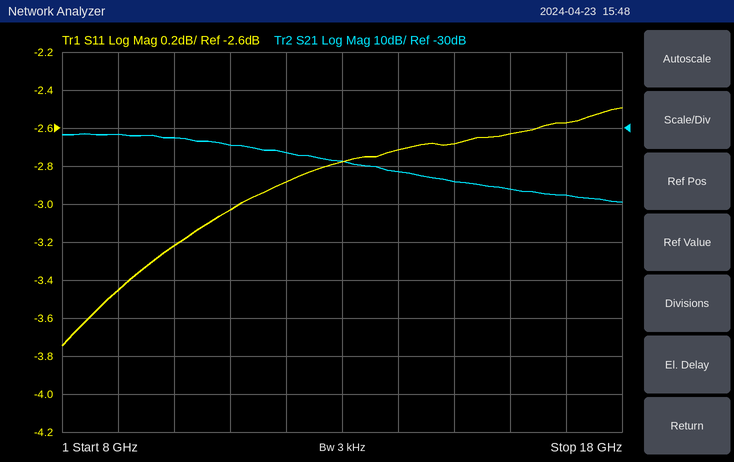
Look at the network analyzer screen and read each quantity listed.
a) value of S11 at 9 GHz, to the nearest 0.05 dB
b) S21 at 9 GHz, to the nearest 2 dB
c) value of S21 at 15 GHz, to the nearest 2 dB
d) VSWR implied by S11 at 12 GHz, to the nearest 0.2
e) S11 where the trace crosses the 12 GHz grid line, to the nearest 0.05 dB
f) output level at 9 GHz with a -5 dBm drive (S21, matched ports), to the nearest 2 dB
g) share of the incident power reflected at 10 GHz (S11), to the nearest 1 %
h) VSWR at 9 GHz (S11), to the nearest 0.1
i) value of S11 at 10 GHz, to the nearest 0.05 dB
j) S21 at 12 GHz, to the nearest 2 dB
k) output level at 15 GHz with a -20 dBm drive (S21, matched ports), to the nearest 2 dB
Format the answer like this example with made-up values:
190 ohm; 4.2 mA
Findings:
-3.45 dB; -32 dB; -44 dB; 6.0; -2.90 dB; -36 dBm; 48 %; 5.1; -3.20 dB; -36 dB; -64 dBm
